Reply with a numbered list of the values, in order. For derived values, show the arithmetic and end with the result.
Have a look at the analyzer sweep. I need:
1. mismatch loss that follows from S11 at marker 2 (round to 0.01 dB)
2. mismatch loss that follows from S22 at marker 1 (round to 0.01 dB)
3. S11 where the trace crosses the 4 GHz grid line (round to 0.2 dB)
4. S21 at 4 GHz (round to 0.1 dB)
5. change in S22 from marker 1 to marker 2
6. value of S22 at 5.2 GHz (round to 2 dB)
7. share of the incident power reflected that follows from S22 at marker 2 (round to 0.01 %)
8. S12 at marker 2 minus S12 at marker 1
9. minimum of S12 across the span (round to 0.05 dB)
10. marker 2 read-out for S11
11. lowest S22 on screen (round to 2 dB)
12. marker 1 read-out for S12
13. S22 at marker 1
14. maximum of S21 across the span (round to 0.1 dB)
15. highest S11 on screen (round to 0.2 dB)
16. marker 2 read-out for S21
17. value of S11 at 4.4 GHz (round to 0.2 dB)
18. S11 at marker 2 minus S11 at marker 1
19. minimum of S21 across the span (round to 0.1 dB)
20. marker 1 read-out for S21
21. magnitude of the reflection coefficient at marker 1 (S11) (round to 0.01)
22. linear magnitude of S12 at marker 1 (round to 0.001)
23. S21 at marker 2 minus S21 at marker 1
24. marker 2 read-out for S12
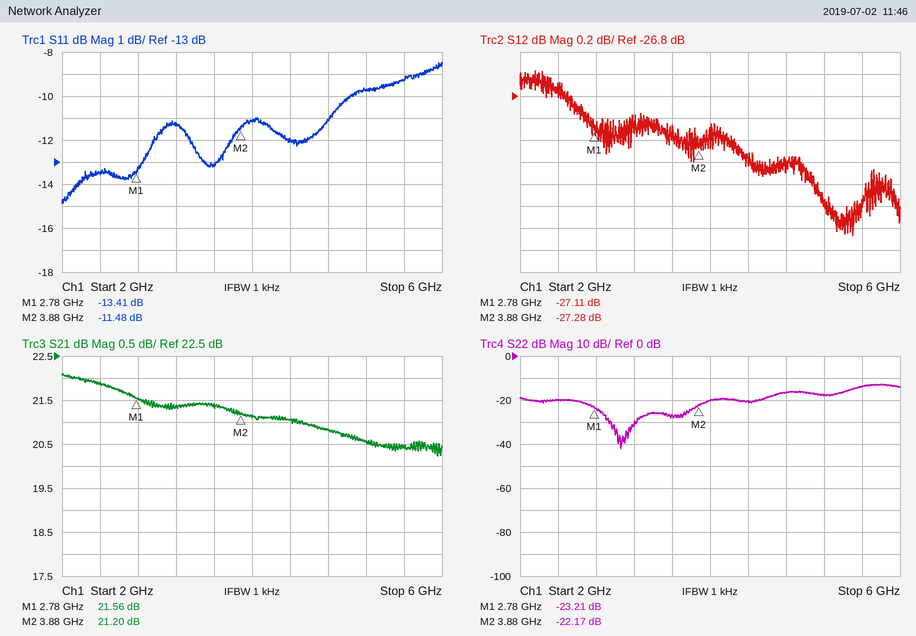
1. −10 log10(1 − 10^(-11.48/10)) ≈ 0.32 dB
2. −10 log10(1 − 10^(-23.21/10)) ≈ 0.02 dB
3. -11.2 dB
4. 21.1 dB
5. -22.17 − (-23.21) = 1.04 dB
6. -18 dB
7. 10^(-22.17/10) ≈ 0.61 %
8. -27.28 − (-27.11) = -0.17 dB
9. -28.05 dB
10. -11.48 dB
11. -42 dB
12. -27.11 dB
13. -23.21 dB
14. 22.1 dB
15. -8.4 dB
16. 21.20 dB
17. -12.0 dB
18. -11.48 − (-13.41) = 1.93 dB
19. 20.2 dB
20. 21.56 dB
21. 10^(-13.41/20) ≈ 0.21
22. 10^(-27.11/20) ≈ 0.044
23. 21.2 − (21.56) = -0.36 dB
24. -27.28 dB
